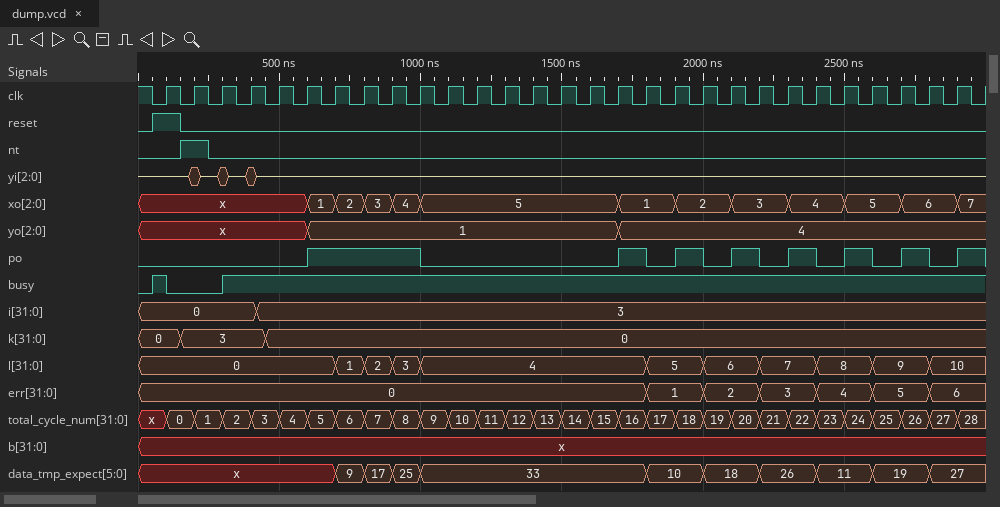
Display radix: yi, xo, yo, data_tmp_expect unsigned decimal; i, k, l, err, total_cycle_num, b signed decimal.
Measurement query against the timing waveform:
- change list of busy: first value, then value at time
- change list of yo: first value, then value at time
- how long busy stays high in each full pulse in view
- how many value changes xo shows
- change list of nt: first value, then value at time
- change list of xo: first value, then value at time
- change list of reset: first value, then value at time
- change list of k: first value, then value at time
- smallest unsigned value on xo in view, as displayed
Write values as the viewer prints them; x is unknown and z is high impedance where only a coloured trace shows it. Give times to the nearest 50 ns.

0, 1 at 50 ns, 0 at 100 ns, 1 at 300 ns
x, 1 at 600 ns, 4 at 1700 ns
50 ns
12
0, 1 at 150 ns, 0 at 250 ns
x, 1 at 600 ns, 2 at 700 ns, 3 at 800 ns, 4 at 900 ns, 5 at 1000 ns, 1 at 1700 ns, 2 at 1900 ns, 3 at 2100 ns, 4 at 2300 ns, 5 at 2500 ns, 6 at 2700 ns, 7 at 2900 ns
0, 1 at 50 ns, 0 at 150 ns
0, 3 at 150 ns, 0 at 450 ns
1
